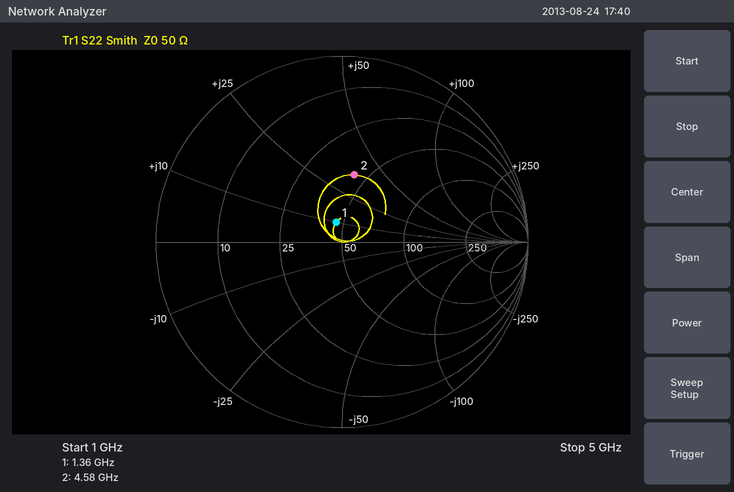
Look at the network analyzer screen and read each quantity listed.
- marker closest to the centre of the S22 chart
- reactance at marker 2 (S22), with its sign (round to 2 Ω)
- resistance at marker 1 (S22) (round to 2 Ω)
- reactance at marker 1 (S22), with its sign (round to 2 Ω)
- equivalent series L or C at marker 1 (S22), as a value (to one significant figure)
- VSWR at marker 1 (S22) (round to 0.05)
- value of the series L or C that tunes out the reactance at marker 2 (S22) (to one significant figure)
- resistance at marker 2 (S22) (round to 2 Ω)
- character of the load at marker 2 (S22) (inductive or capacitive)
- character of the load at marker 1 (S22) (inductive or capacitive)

marker 1
+36 Ω
46 Ω
+10 Ω
1 nH
1.25
1.0 pF
44 Ω
inductive
inductive
